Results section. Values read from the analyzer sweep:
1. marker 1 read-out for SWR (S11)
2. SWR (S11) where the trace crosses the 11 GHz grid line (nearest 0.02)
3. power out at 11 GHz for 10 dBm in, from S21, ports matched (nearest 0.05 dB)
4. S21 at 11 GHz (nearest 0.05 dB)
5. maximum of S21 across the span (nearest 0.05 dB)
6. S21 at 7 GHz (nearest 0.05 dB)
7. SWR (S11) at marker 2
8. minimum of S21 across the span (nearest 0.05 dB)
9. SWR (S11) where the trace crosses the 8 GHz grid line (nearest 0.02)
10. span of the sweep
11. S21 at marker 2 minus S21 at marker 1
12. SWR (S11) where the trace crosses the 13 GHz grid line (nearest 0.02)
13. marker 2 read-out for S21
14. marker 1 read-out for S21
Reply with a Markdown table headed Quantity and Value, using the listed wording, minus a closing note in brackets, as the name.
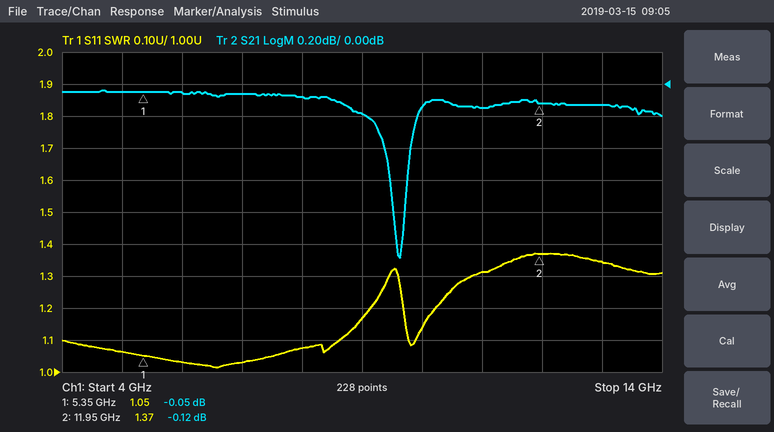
| Quantity | Value |
|---|---|
| marker 1 read-out for SWR | 1.05 |
| SWR (S11) where the trace crosses the 11 GHz grid line | 1.32 |
| power out at 11 GHz for 10 dBm in, from S21, ports matched | 9.85 dBm |
| S21 at 11 GHz | -0.15 dB |
| maximum of S21 across the span | -0.05 dB |
| S21 at 7 GHz | -0.05 dB |
| SWR (S11) at marker 2 | 1.37 |
| minimum of S21 across the span | -1.10 dB |
| SWR (S11) where the trace crosses the 8 GHz grid line | 1.08 |
| span of the sweep | 10 GHz |
| S21 at marker 2 minus S21 at marker 1 | -0.07 dB |
| SWR (S11) where the trace crosses the 13 GHz grid line | 1.34 |
| marker 2 read-out for S21 | -0.12 dB |
| marker 1 read-out for S21 | -0.05 dB |
